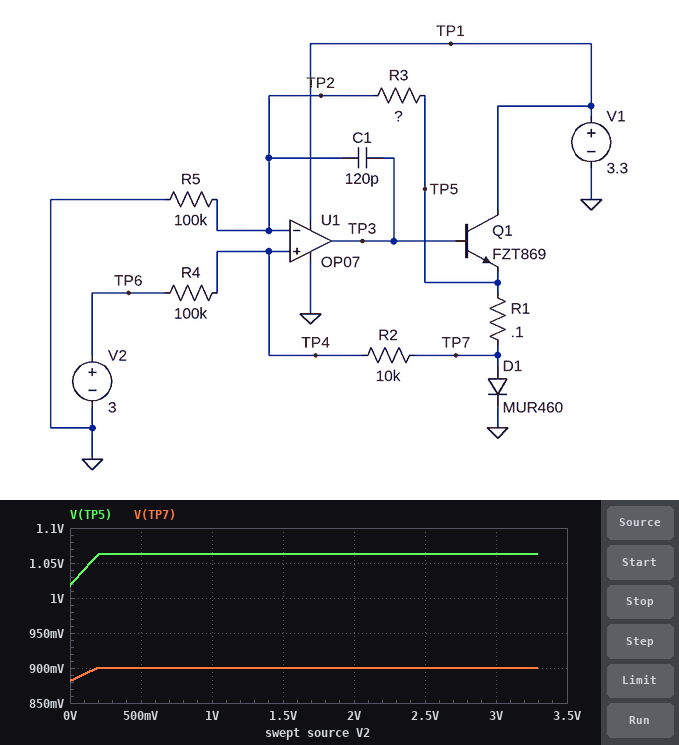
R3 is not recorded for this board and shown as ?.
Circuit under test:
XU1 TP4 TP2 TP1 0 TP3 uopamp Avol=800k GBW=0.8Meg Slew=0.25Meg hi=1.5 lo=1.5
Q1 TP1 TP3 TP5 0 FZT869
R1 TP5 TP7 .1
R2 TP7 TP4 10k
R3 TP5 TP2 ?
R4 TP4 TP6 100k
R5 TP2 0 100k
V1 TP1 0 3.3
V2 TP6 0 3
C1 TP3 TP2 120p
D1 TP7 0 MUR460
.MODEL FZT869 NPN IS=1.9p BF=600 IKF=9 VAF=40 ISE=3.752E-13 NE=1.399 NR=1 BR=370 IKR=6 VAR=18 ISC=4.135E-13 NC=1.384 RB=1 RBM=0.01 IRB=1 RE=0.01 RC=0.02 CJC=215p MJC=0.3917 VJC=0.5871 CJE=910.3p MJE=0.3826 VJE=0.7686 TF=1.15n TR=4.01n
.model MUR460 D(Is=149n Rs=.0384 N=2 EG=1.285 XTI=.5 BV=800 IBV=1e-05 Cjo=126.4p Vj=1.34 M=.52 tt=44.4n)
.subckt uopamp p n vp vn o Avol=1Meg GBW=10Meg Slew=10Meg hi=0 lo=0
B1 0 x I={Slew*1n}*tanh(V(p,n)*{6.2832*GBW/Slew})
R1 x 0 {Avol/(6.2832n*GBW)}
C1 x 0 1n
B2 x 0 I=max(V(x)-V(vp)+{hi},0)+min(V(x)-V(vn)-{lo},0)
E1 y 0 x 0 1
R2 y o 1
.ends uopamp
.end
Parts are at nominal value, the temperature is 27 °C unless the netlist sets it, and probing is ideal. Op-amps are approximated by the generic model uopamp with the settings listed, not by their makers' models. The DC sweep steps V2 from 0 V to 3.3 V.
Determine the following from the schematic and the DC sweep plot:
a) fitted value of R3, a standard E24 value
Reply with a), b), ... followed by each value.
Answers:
a) 27 kΩ
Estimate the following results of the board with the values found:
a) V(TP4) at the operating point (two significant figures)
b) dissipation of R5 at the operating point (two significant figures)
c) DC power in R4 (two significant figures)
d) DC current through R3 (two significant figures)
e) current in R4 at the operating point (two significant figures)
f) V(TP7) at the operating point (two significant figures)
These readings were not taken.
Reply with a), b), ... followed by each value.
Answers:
a) 1.1 V
b) 7.0 µW
c) 36 µW
d) 8.4 µA
e) 19 µA
f) 900 mV
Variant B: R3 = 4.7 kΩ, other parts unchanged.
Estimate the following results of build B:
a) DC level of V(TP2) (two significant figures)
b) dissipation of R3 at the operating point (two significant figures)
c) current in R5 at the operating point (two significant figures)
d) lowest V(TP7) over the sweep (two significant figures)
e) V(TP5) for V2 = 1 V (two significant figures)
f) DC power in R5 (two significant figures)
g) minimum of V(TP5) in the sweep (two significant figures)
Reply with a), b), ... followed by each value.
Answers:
a) 1.0 V
b) 480 nW
c) 10 µA
d) 780 mV
e) 860 mV
f) 10 µW
g) 820 mV
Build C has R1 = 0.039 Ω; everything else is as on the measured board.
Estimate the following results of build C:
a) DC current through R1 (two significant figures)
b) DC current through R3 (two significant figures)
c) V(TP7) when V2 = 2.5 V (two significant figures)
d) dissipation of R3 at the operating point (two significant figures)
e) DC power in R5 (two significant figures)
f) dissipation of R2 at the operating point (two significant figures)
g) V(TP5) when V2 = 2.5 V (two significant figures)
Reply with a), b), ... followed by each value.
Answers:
a) 2.4 A
b) 8.2 µA
c) 950 mV
d) 1.8 µW
e) 6.7 µW
f) 3.5 µW
g) 1.0 V
